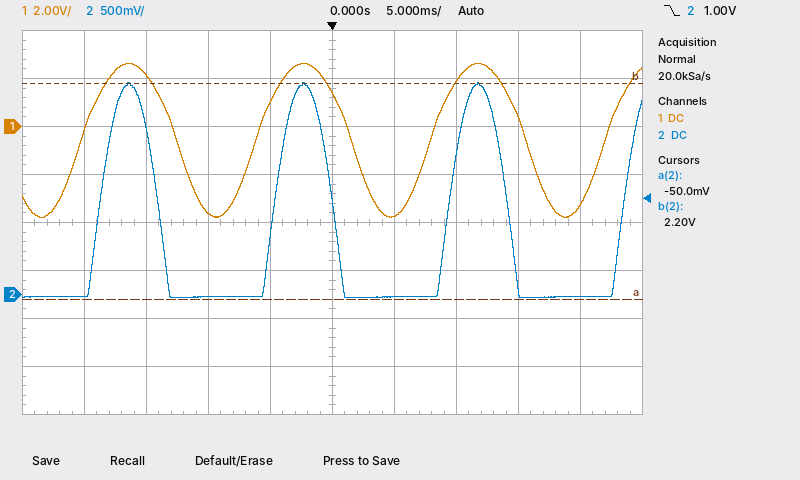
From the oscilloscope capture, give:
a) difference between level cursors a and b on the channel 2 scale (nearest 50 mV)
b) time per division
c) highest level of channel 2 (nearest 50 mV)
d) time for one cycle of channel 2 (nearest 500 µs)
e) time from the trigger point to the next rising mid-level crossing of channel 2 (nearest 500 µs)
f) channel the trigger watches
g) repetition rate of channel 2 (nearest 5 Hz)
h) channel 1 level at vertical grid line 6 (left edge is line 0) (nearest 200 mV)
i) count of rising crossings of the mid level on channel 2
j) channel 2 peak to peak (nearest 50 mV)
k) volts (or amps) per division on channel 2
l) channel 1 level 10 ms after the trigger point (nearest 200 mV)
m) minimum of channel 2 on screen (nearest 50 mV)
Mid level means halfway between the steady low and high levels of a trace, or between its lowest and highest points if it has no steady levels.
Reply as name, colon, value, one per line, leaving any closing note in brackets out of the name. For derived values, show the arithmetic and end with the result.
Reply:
difference between level cursors a and b on the channel 2 scale: 2.25 V
time per division: 5 ms
highest level of channel 2: 2.20 V
time for one cycle of channel 2: 14.0 ms
time from the trigger point to the next rising mid-level crossing of channel 2: 9.5 ms
channel the trigger watches: channel 2
repetition rate of channel 2: 1 / 14.0 ms ≈ 71.4 Hz, so 70 Hz to the nearest 5 Hz
channel 1 level at vertical grid line 6 (left edge is line 0): -3.8 V
count of rising crossings of the mid level on channel 2: 4
channel 2 peak to peak: 2.20 V − (-50 mV) = 2.25 V
volts (or amps) per division on channel 2: 500 mV
channel 1 level 10 ms after the trigger point: 1.8 V
minimum of channel 2 on screen: -50 mV
